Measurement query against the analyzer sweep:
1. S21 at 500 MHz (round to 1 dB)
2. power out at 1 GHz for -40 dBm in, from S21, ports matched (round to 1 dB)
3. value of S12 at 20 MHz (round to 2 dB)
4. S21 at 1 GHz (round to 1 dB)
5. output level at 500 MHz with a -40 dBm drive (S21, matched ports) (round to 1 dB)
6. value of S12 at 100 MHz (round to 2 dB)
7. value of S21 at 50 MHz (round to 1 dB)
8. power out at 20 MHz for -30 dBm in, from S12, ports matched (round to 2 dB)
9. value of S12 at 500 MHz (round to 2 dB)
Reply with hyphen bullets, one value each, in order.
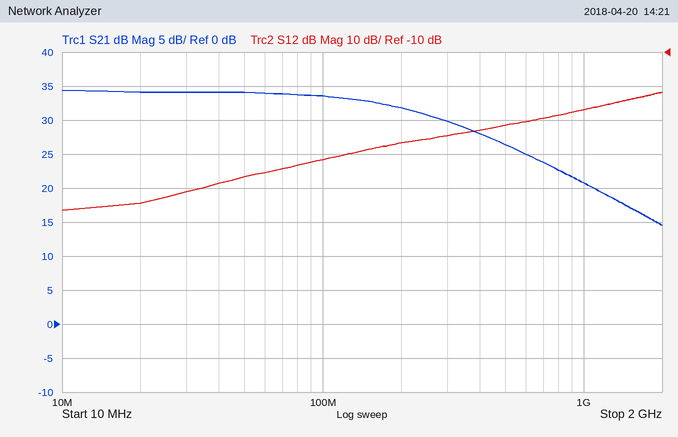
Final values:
- 26 dB
- -19 dBm
- -54 dB
- 21 dB
- -14 dBm
- -42 dB
- 34 dB
- -84 dBm
- -32 dB
